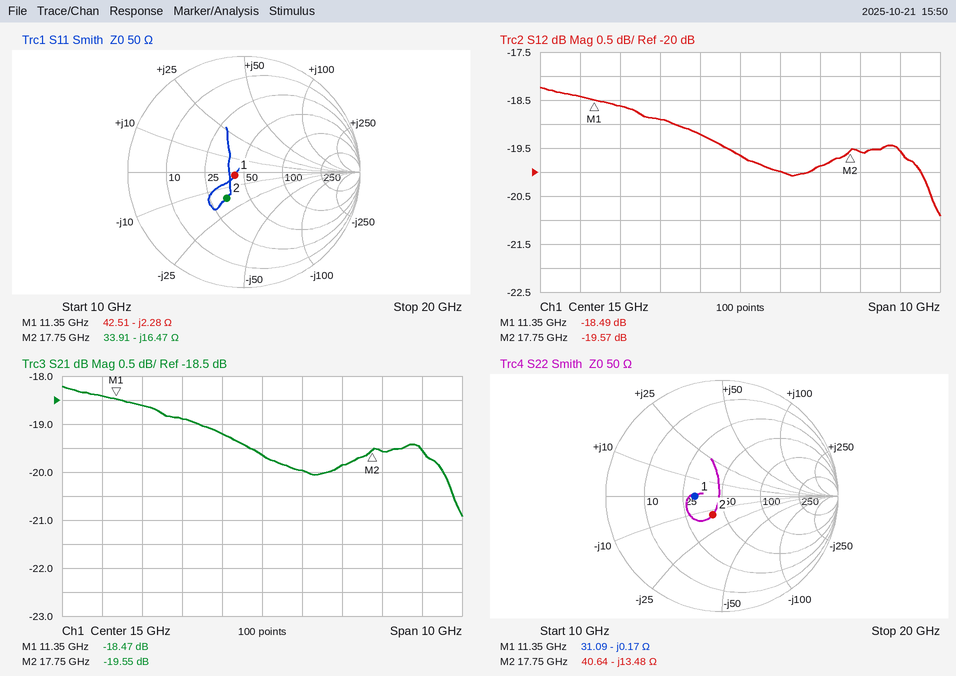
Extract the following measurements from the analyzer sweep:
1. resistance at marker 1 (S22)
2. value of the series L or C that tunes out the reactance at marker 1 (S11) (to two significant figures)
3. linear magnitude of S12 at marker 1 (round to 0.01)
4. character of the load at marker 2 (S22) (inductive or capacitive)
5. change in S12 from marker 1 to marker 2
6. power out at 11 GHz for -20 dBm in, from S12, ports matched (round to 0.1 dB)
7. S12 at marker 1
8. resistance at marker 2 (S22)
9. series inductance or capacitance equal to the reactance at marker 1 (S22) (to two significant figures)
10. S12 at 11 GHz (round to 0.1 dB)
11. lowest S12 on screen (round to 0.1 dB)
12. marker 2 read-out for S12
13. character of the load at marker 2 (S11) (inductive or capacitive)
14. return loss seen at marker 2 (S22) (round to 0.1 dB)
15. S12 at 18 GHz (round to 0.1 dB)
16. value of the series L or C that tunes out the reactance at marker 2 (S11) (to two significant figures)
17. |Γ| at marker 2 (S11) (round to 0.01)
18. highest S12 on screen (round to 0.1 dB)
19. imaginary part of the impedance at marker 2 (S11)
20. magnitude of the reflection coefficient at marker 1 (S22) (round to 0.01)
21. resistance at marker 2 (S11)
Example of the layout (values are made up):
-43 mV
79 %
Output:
31.09 Ω
32 pH
0.12
capacitive
-1.08 dB
-38.4 dBm
-18.49 dB
40.64 Ω
82 pF
-18.4 dB
-20.9 dB
-19.57 dB
capacitive
14.9 dB
-19.6 dB
150 pH
0.27
-18.2 dB
-16.47 Ω
0.23
33.91 Ω
